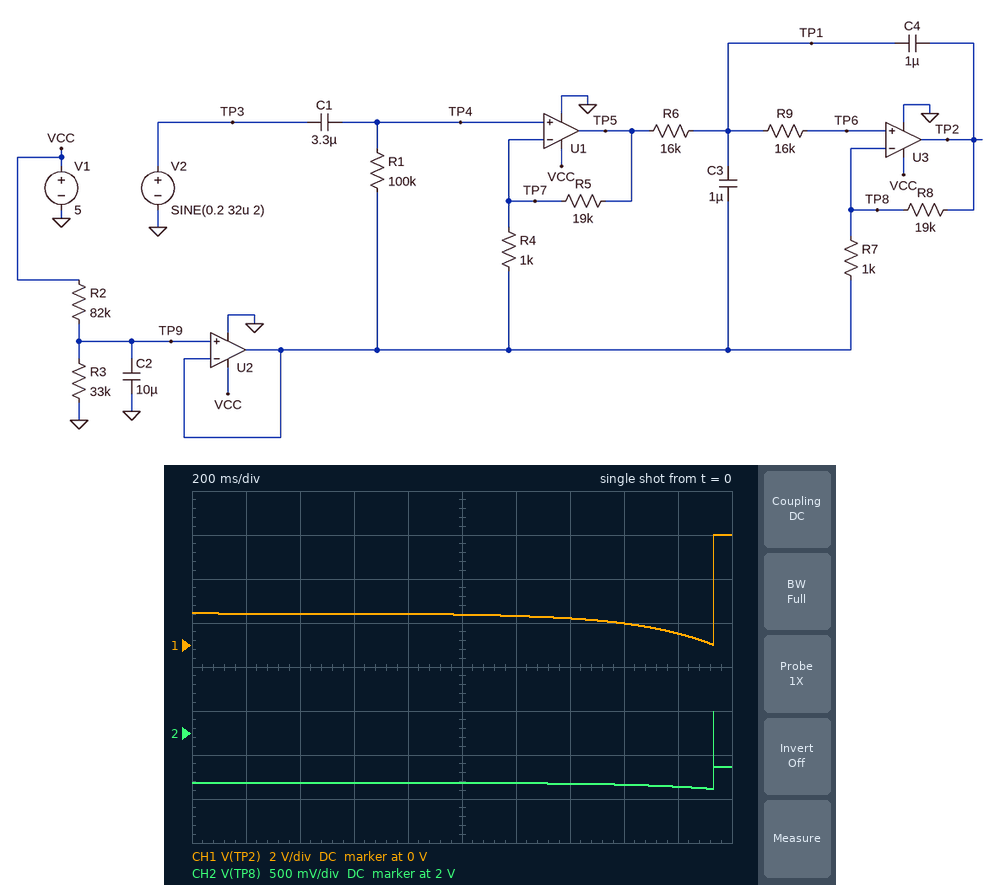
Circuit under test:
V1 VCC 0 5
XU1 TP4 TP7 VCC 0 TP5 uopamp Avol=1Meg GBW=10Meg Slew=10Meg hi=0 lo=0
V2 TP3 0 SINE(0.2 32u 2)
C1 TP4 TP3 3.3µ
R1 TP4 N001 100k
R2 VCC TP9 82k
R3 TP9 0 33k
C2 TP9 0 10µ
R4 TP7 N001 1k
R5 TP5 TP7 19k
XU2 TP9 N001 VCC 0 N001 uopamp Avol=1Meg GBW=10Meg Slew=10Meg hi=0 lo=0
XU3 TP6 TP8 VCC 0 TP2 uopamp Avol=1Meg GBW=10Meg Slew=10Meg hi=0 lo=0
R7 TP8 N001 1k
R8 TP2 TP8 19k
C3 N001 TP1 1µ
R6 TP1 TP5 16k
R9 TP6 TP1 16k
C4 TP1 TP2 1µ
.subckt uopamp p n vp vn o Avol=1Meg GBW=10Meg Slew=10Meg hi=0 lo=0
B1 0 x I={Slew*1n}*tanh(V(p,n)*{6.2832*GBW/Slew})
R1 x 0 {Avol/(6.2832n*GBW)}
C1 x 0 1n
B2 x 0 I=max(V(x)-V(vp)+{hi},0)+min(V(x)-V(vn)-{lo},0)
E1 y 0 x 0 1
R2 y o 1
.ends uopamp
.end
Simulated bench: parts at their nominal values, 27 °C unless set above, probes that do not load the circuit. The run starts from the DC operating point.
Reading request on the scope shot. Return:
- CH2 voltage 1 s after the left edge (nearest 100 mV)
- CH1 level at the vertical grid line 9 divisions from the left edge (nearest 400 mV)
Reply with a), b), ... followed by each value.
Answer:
a) 1.4 V
b) 400 mV
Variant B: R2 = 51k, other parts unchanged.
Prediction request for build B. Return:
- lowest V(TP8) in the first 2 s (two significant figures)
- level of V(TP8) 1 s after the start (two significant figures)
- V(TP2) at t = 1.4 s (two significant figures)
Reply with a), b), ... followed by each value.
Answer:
a) 1.9 V
b) 2.0 V
c) 1.7 V
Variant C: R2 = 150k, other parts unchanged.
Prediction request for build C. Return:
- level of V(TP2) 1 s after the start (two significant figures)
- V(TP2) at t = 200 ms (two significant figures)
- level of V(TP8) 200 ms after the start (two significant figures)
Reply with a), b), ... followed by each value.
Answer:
a) 850 mV
b) 890 mV
c) 900 mV
